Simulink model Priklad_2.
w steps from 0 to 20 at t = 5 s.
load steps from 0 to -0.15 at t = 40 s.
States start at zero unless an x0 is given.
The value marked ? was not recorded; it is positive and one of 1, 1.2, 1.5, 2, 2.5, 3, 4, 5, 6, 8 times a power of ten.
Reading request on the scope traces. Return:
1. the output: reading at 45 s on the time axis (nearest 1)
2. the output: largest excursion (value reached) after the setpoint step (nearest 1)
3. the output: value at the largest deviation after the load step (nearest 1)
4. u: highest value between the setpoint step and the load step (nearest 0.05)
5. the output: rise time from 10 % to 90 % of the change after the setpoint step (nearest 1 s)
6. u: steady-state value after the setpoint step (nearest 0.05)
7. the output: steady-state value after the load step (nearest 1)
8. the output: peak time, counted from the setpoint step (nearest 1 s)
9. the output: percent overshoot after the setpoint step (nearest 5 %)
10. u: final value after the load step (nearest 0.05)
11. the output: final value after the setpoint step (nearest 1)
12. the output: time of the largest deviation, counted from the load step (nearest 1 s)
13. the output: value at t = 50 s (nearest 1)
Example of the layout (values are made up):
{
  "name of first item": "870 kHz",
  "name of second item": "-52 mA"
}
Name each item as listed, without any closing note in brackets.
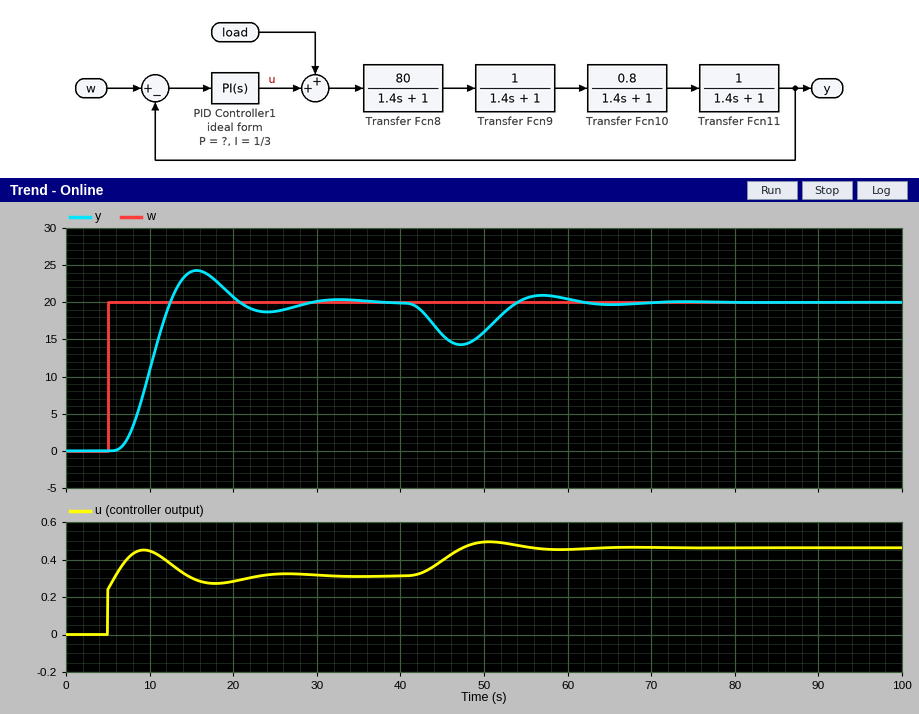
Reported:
{
  "the output: reading at 45 s on the time axis": "16",
  "the output: largest excursion (value reached) after the setpoint step": "24",
  "the output: value at the largest deviation after the load step": "14",
  "u: highest value between the setpoint step and the load step": "0.45",
  "the output: rise time from 10 % to 90 % of the change after the setpoint step": "4 s",
  "u: steady-state value after the setpoint step": "0.30",
  "the output: steady-state value after the load step": "20",
  "the output: peak time, counted from the setpoint step": "11 s",
  "the output: percent overshoot after the setpoint step": "20 %",
  "u: final value after the load step": "0.45",
  "the output: final value after the setpoint step": "20",
  "the output: time of the largest deviation, counted from the load step": "7 s",
  "the output: value at t = 50 s": "16"
}
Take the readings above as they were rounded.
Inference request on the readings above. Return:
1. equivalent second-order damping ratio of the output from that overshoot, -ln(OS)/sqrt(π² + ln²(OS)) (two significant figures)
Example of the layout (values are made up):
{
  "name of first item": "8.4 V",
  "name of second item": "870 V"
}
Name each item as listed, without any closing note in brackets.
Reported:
{
  "equivalent second-order damping ratio of the output from that overshoot, -ln(OS)/sqrt(π² + ln²(OS))": "0.46"
}
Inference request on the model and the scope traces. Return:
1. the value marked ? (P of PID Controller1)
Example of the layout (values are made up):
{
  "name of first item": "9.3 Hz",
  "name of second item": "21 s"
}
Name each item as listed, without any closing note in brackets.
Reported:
{
  "the value marked ?": "0.012"
}
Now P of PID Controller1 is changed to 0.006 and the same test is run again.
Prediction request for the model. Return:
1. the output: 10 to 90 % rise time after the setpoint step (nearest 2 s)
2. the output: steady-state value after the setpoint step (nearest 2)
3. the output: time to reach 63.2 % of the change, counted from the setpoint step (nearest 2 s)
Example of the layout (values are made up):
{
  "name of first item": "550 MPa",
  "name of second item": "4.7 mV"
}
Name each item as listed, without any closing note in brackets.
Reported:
{
  "the output: 10 to 90 % rise time after the setpoint step": "10 s",
  "the output: steady-state value after the setpoint step": "20",
  "the output: time to reach 63.2 % of the change, counted from the setpoint step": "8 s"
}
